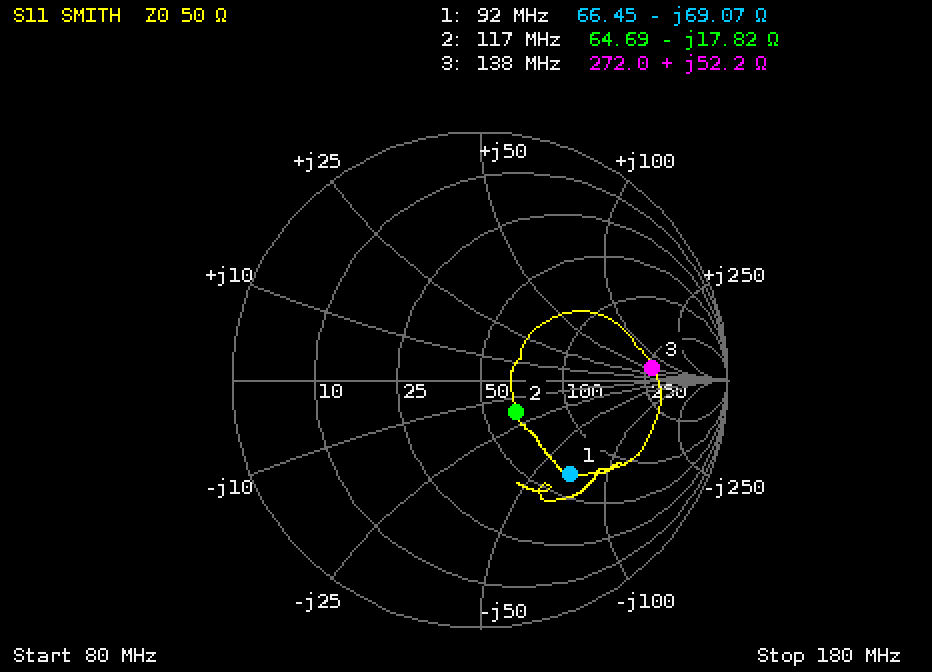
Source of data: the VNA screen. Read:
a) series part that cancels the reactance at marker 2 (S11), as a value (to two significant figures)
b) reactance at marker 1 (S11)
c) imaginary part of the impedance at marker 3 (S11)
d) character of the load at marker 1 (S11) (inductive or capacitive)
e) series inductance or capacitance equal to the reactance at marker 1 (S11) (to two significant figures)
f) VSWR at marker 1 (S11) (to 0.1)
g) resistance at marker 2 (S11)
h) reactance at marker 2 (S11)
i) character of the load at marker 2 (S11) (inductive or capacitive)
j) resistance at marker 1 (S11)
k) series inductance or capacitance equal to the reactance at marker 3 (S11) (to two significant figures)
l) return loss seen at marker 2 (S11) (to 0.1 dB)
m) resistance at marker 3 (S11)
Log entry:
24 nH
-69.07 Ω
+52.2 Ω
capacitive
25 pF
3.2
64.69 Ω
-17.82 Ω
capacitive
66.45 Ω
60 nH
14.0 dB
272.0 Ω
